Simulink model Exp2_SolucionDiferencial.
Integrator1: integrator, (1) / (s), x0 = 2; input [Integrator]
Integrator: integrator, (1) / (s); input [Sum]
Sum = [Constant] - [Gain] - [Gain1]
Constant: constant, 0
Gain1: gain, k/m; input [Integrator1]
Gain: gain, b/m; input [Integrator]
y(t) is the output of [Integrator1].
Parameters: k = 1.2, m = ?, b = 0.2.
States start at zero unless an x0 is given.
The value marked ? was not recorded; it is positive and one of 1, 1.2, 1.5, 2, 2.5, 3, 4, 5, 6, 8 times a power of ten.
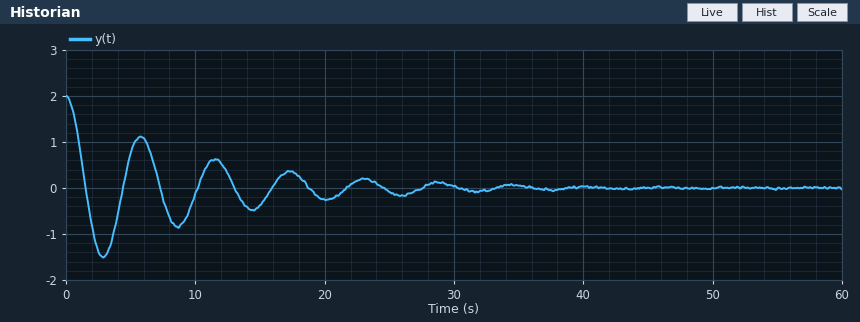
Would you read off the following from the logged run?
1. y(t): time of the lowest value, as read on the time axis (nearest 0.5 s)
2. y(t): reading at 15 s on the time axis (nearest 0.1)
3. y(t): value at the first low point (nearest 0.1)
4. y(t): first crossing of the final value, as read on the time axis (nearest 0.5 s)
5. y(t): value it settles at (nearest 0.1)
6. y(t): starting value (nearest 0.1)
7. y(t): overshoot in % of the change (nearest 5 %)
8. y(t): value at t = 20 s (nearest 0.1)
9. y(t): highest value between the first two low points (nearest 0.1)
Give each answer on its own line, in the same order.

3.0 s
-0.4
-1.5
1.5 s
0.0
2.0
75 %
-0.3
1.1
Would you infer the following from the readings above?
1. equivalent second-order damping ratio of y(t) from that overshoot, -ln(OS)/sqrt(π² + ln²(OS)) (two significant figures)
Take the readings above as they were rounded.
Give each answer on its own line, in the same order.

0.091
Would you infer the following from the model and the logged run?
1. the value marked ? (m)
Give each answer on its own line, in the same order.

1
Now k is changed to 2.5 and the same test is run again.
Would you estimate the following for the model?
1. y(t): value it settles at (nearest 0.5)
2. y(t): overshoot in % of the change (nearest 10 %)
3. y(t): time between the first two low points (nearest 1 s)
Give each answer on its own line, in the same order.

0.0
80 %
4 s
